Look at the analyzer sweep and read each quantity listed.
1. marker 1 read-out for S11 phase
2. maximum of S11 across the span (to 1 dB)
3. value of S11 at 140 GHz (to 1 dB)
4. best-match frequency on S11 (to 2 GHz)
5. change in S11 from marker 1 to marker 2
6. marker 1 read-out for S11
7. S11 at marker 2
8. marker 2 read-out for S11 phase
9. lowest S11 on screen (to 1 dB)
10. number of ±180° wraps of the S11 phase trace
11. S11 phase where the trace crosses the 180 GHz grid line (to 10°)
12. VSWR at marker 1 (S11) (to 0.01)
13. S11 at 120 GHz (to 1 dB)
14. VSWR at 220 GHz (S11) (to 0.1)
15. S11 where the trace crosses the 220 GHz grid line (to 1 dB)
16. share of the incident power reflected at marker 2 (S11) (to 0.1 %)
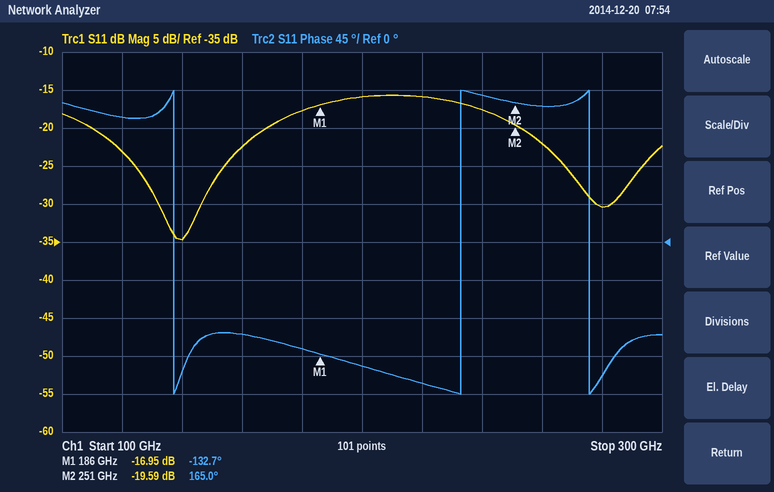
-132.7°
-16 dB
-35 dB
140 GHz
-2.64 dB
-16.95 dB
-19.59 dB
165.0°
-35 dB
3
-130°
1.33
-23 dB
1.4
-16 dB
1.1 %
